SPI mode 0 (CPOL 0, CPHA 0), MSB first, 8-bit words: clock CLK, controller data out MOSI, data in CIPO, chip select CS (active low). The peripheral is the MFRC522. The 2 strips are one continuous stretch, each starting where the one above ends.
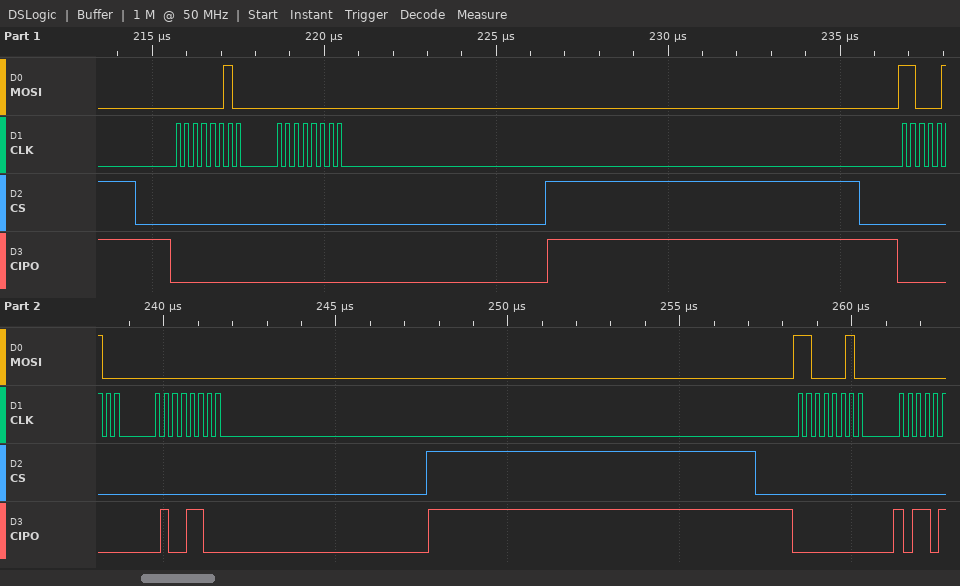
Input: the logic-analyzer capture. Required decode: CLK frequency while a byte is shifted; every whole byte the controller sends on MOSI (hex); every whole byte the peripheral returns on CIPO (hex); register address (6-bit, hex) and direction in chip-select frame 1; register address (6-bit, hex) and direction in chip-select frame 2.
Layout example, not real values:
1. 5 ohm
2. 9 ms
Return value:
1. 4 MHz
2. 02 00 C4 00 C2
3. 00 00 00 4C 00
4. 0x01 write
5. 0x22 read
